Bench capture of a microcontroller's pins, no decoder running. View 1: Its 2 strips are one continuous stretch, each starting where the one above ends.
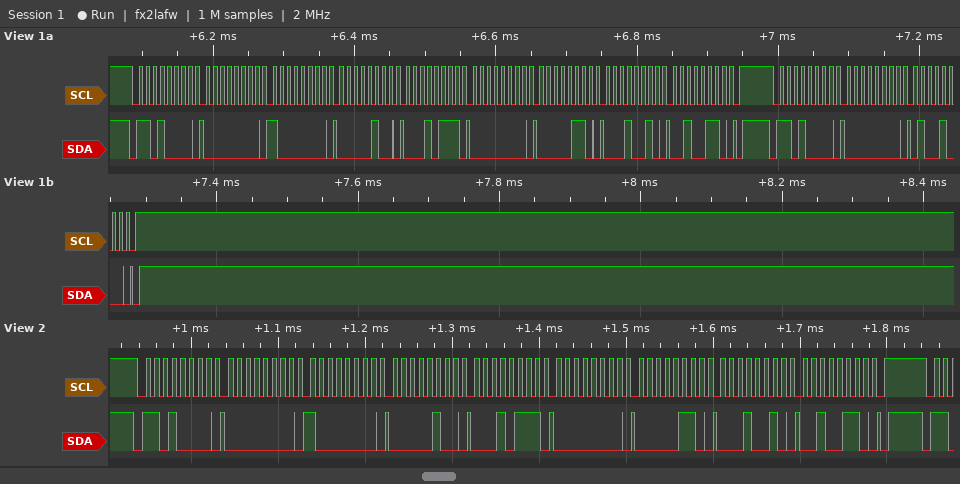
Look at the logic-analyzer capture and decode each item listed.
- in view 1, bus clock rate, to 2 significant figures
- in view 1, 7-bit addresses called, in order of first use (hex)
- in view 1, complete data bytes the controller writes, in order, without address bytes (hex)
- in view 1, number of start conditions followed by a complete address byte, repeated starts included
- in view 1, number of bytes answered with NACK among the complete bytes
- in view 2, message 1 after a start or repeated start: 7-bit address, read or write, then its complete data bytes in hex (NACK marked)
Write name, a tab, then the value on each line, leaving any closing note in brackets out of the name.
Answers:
in view 1, bus clock rate, to 2 significant figures	100 kHz
in view 1, 7-bit addresses called, in order of first use	0x68
in view 1, complete data bytes the controller writes, in order, without address bytes	00 80 04 17 00 06 12 26 00 48
in view 1, number of start conditions followed by a complete address byte, repeated starts included	2
in view 1, number of bytes answered with NACK among the complete bytes	0
in view 2, message 1 after a start or repeated start: 7-bit address, read or write, then its complete data bytes in hex	0x68 write: 00 80 04 17 00 06 12 26
